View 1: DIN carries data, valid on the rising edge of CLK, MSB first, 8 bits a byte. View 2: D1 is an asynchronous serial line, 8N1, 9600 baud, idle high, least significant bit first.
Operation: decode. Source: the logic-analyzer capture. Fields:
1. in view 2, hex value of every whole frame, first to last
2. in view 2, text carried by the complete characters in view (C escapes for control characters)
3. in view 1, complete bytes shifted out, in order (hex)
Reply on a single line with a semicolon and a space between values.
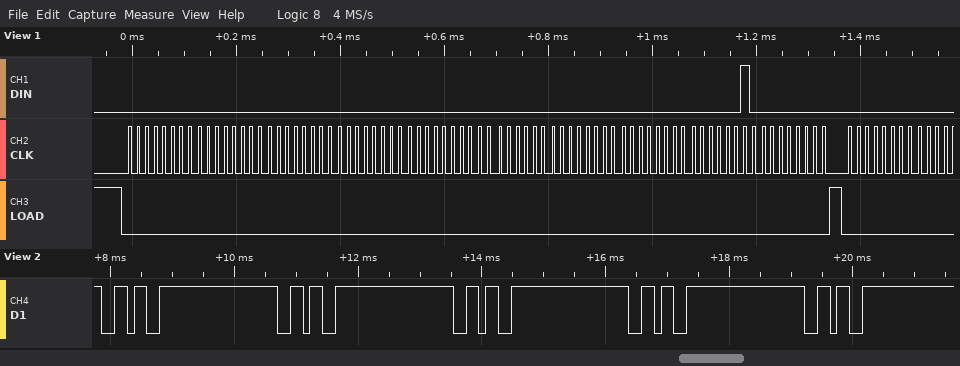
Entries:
36 36 36 36 36; "66666"; 00 00 00 00 00 00 00 00 02 00 00
